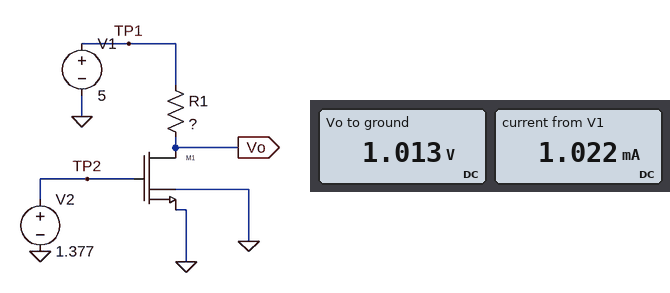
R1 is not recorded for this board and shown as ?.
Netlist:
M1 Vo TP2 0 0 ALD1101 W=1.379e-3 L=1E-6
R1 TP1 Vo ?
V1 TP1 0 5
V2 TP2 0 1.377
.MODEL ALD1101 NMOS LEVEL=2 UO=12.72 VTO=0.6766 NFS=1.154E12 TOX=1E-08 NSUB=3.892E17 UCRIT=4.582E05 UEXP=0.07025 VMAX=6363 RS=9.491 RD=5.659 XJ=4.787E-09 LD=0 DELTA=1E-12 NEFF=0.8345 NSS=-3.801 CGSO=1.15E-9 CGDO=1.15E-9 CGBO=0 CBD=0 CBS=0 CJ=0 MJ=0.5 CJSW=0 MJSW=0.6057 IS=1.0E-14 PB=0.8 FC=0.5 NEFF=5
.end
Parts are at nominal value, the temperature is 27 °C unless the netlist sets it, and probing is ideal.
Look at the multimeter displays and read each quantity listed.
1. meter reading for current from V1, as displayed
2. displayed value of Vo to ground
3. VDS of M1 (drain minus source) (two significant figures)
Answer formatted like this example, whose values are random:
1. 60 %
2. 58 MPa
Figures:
1. 1.022 mA
2. 1.013 V
3. 1.0 V
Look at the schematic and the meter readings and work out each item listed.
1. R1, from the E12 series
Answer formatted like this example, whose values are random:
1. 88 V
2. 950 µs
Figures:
1. 3.9 kΩ
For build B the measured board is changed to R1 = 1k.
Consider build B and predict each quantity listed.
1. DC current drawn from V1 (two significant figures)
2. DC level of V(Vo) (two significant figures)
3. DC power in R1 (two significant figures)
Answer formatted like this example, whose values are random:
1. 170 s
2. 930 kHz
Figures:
1. 1.1 mA
2. 3.9 V
3. 1.1 mW
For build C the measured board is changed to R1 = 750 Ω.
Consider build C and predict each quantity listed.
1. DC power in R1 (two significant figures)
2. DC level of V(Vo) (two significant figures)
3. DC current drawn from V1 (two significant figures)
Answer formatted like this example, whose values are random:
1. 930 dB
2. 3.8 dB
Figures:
1. 850 µW
2. 4.2 V
3. 1.1 mA
